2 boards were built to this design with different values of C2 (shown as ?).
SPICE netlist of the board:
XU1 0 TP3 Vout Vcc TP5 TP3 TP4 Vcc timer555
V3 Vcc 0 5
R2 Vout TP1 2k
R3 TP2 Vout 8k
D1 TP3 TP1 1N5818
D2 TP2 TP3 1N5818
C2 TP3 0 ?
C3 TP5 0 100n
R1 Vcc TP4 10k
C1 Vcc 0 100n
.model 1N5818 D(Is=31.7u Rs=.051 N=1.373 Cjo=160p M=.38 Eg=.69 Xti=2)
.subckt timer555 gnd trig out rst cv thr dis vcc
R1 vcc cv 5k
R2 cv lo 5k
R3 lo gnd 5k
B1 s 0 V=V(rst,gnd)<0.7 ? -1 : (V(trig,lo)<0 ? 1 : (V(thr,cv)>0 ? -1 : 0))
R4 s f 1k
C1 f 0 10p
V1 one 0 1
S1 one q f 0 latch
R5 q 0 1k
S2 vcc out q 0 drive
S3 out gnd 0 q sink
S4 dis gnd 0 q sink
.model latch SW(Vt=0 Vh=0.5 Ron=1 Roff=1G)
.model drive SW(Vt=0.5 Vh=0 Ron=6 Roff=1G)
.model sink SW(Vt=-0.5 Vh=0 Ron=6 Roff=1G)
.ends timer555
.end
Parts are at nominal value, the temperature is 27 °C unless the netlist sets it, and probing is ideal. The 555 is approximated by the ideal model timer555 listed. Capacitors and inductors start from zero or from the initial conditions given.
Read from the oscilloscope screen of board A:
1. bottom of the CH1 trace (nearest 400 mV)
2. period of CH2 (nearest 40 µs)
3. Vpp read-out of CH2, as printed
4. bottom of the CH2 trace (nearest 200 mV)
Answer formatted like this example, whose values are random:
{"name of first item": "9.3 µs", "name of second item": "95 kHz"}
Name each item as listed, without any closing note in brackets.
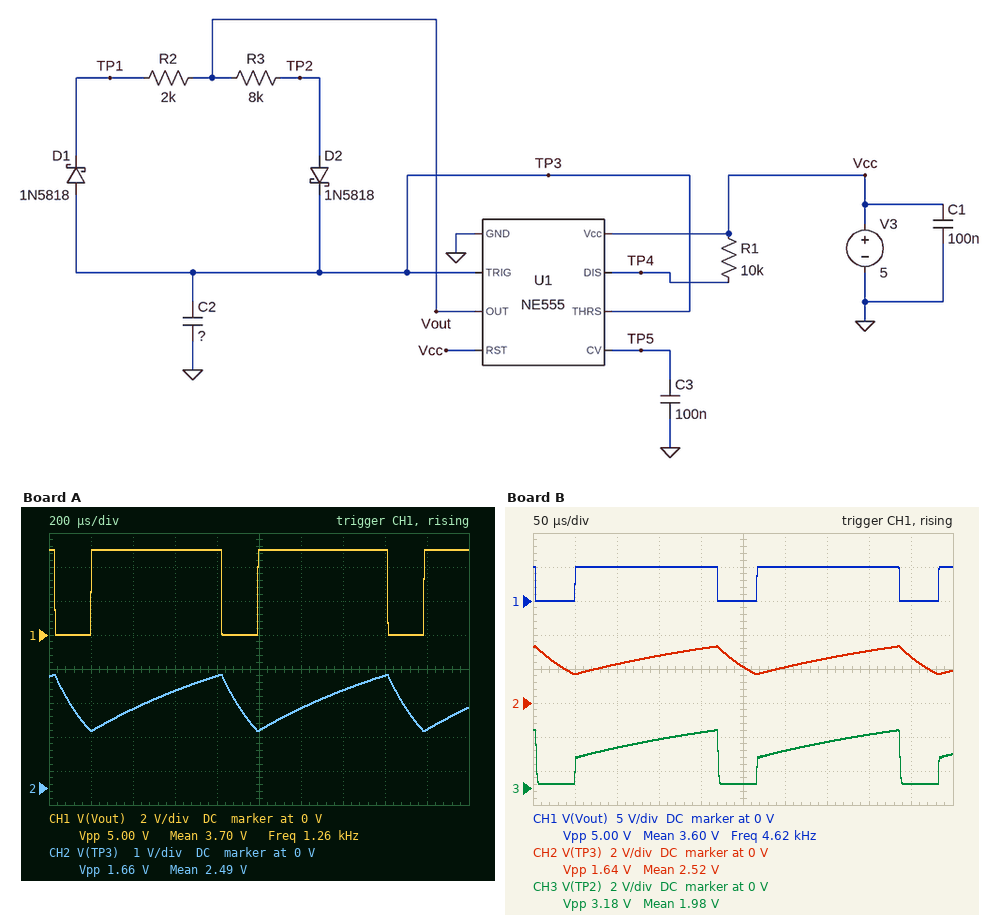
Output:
{"bottom of the CH1 trace": "0 V", "period of CH2": "800 µs", "Vpp read-out of CH2, as printed": "1.66 V", "bottom of the CH2 trace": "1.6 V"}
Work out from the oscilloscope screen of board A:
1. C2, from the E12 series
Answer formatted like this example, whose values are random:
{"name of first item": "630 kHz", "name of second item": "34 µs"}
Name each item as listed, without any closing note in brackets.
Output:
{"C2, from the E12 series": "120 nF"}
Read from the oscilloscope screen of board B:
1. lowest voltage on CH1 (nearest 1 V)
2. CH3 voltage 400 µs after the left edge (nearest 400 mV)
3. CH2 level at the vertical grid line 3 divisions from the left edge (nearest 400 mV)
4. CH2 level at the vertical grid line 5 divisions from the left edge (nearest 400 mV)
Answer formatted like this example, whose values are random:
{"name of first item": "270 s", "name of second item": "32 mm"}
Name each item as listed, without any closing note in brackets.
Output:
{"lowest voltage on CH1": "0 V", "CH3 voltage 400 µs after the left edge": "3.2 V", "CH2 level at the vertical grid line 3 divisions from the left edge": "2.8 V", "CH2 level at the vertical grid line 5 divisions from the left edge": "2.0 V"}
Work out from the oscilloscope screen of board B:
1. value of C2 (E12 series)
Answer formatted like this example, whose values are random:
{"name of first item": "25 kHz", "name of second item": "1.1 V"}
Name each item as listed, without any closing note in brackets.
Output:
{"value of C2": "33 nF"}
